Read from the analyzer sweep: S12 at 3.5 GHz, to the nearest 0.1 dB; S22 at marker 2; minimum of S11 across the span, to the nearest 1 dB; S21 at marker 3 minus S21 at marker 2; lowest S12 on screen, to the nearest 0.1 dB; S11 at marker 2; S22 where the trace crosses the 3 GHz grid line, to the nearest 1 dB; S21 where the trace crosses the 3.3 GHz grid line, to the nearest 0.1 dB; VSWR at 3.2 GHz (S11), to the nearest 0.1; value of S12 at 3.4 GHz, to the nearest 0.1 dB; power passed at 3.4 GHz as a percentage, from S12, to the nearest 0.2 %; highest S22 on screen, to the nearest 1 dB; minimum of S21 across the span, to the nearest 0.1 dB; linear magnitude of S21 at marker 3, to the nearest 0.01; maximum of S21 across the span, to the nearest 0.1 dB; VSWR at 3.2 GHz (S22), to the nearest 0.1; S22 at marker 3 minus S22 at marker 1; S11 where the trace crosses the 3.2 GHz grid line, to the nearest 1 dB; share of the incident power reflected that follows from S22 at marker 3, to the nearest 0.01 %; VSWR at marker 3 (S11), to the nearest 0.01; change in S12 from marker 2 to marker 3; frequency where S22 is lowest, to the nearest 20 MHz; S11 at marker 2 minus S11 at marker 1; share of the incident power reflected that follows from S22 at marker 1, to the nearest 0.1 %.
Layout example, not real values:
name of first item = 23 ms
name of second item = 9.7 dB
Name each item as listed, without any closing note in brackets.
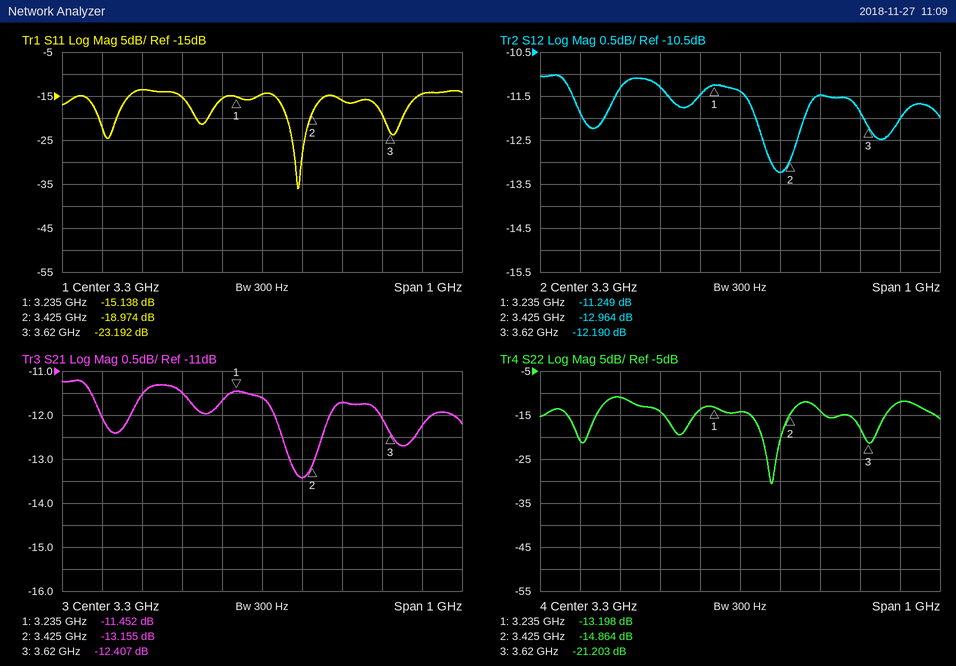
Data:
S12 at 3.5 GHz, to the nearest 0.1 dB = -11.5 dB
S22 at marker 2 = -14.864 dB
minimum of S11 across the span, to the nearest 1 dB = -36 dB
S21 at marker 3 minus S21 at marker 2 = 0.748 dB
lowest S12 on screen, to the nearest 0.1 dB = -13.2 dB
S11 at marker 2 = -18.974 dB
S22 where the trace crosses the 3 GHz grid line, to the nearest 1 dB = -11 dB
S21 where the trace crosses the 3.3 GHz grid line, to the nearest 0.1 dB = -11.6 dB
VSWR at 3.2 GHz (S11), to the nearest 0.1 = 1.4
value of S12 at 3.4 GHz, to the nearest 0.1 dB = -13.2 dB
power passed at 3.4 GHz as a percentage, from S12, to the nearest 0.2 % = 4.8 %
highest S22 on screen, to the nearest 1 dB = -11 dB
minimum of S21 across the span, to the nearest 0.1 dB = -13.4 dB
linear magnitude of S21 at marker 3, to the nearest 0.01 = 0.24
maximum of S21 across the span, to the nearest 0.1 dB = -11.2 dB
VSWR at 3.2 GHz (S22), to the nearest 0.1 = 1.5
S22 at marker 3 minus S22 at marker 1 = -8.005 dB
S11 where the trace crosses the 3.2 GHz grid line, to the nearest 1 dB = -16 dB
share of the incident power reflected that follows from S22 at marker 3, to the nearest 0.01 % = 0.76 %
VSWR at marker 3 (S11), to the nearest 0.01 = 1.15
change in S12 from marker 2 to marker 3 = 0.774 dB
frequency where S22 is lowest, to the nearest 20 MHz = 3.38 GHz
S11 at marker 2 minus S11 at marker 1 = -3.836 dB
share of the incident power reflected that follows from S22 at marker 1, to the nearest 0.1 % = 4.8 %
